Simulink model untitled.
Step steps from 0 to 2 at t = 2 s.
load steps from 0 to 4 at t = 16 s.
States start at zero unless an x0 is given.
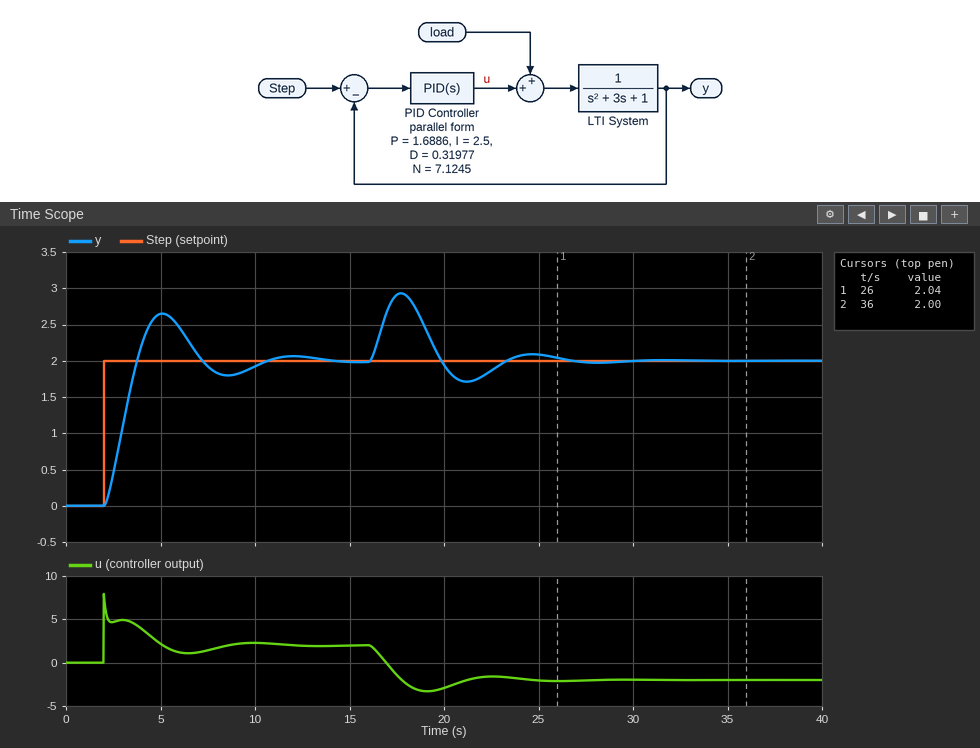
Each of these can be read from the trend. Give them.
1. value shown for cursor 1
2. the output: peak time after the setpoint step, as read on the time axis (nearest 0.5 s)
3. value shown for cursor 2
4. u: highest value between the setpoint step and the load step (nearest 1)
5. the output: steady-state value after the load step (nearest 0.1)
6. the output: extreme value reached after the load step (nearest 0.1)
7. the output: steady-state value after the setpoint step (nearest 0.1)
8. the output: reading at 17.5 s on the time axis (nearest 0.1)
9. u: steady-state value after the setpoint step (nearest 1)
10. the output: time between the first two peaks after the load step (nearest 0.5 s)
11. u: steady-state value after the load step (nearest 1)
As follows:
2.04
5.0 s
2.00
8
2.0
2.9
2.0
2.9
2
7.0 s
-2
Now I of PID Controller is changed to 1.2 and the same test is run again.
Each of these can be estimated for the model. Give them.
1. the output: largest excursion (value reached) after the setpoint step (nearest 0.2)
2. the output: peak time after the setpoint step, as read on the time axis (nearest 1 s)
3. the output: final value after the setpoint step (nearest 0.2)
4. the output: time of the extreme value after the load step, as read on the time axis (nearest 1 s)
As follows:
2.2
6 s
2.0
18 s
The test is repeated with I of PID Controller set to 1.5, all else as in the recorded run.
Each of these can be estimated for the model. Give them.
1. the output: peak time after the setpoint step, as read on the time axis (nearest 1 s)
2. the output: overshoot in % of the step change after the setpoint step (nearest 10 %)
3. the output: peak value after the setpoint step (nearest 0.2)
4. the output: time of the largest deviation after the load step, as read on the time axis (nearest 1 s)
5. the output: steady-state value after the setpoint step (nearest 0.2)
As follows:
6 s
20 %
2.4
18 s
2.0
